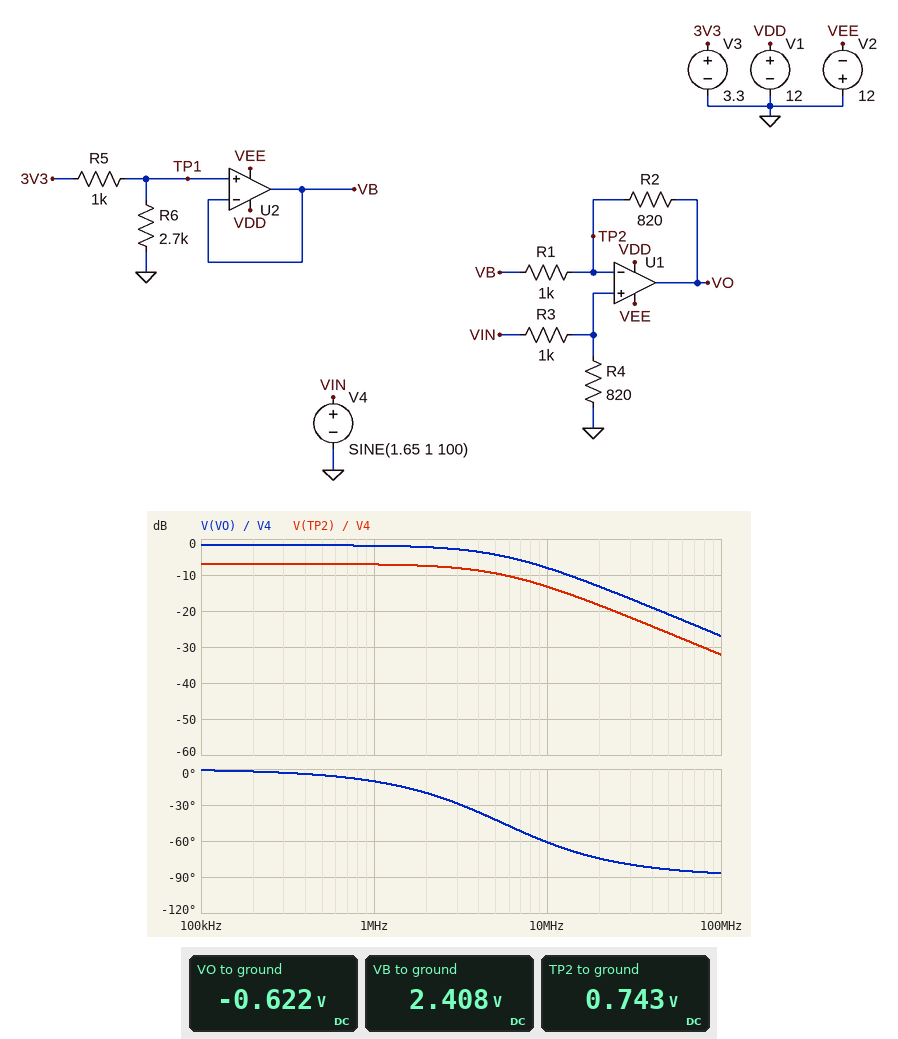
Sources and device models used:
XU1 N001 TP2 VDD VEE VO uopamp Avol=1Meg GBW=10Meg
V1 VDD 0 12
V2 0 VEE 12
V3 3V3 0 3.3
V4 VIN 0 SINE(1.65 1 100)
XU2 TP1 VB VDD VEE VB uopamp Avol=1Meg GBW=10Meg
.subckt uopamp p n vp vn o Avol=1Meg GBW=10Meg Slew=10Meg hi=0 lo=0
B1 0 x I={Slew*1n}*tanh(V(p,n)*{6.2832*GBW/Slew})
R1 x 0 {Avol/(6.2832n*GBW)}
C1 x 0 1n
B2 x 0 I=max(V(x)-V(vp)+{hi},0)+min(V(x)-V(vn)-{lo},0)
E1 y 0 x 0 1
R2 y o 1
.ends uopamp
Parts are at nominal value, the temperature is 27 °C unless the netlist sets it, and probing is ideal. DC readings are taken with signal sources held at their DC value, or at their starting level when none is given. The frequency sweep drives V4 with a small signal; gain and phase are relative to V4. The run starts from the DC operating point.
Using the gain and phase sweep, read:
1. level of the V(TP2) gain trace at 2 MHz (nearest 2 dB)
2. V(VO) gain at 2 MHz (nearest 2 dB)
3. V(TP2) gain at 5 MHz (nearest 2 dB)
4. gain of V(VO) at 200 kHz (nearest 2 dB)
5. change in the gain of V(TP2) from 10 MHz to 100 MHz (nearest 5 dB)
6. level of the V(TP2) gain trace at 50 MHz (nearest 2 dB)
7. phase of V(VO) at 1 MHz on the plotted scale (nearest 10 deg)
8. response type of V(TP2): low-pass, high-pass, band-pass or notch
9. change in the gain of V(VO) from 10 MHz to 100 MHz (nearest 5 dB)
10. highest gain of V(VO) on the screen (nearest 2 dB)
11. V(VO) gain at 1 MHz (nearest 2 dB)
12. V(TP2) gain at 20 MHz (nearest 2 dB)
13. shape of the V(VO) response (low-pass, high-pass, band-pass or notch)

-8 dB
-2 dB
-10 dB
-2 dB
-20 dB
-26 dB
-10 deg
low-pass
-20 dB
-2 dB
-2 dB
-18 dB
low-pass
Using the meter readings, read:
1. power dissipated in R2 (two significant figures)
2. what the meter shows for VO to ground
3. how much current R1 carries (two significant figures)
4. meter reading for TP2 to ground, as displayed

2.3 mW
-0.622 V
1.7 mA
0.743 V
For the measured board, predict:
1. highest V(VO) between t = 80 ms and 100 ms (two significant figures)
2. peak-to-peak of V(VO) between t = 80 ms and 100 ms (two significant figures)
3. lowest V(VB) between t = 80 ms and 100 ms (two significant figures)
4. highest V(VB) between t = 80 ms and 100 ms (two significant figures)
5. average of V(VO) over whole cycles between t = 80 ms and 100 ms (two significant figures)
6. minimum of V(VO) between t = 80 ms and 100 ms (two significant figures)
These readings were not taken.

200 mV
1.6 V
2.4 V
2.4 V
-620 mV
-1.4 V
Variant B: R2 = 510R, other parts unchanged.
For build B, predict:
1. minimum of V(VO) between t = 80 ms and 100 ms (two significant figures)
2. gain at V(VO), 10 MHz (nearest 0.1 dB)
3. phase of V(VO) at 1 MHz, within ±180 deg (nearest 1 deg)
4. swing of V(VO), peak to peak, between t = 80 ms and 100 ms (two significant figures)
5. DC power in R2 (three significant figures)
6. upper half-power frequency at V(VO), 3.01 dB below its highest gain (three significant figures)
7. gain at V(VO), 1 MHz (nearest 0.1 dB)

-790 mV
-8.5 dB
-9 deg
1.4 V
1.41 mW
6.62 MHz
-3.4 dB
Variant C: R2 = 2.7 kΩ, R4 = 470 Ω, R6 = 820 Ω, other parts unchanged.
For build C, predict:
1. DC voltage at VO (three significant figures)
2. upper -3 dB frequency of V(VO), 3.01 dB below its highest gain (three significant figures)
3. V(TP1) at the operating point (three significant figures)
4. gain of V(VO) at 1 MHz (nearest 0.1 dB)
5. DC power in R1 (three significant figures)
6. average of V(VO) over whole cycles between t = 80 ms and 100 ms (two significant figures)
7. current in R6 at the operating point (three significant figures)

-2.06 V
2.70 MHz
1.49 V
0.9 dB
920 µW
-2.1 V
1.81 mA
